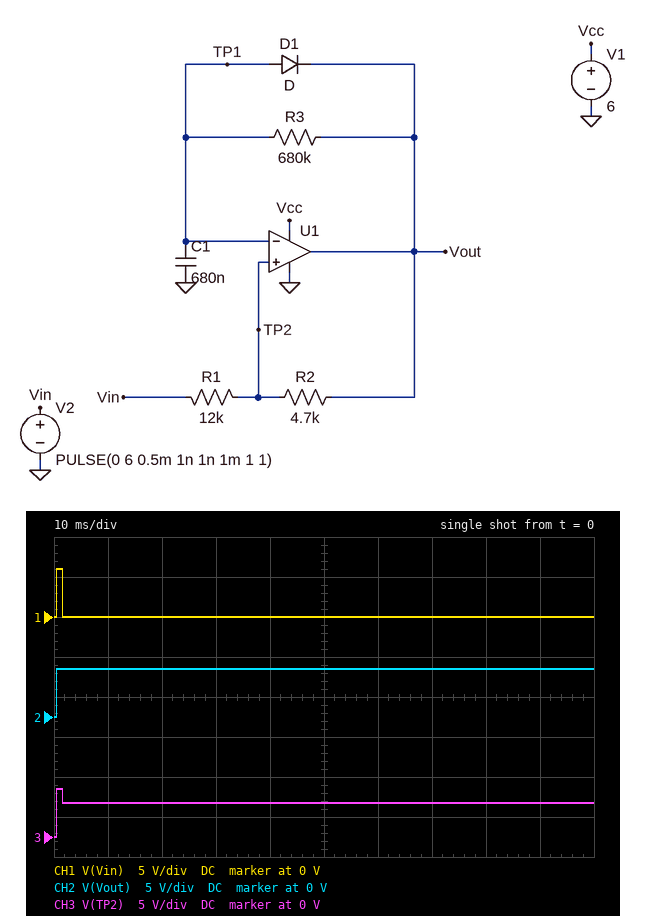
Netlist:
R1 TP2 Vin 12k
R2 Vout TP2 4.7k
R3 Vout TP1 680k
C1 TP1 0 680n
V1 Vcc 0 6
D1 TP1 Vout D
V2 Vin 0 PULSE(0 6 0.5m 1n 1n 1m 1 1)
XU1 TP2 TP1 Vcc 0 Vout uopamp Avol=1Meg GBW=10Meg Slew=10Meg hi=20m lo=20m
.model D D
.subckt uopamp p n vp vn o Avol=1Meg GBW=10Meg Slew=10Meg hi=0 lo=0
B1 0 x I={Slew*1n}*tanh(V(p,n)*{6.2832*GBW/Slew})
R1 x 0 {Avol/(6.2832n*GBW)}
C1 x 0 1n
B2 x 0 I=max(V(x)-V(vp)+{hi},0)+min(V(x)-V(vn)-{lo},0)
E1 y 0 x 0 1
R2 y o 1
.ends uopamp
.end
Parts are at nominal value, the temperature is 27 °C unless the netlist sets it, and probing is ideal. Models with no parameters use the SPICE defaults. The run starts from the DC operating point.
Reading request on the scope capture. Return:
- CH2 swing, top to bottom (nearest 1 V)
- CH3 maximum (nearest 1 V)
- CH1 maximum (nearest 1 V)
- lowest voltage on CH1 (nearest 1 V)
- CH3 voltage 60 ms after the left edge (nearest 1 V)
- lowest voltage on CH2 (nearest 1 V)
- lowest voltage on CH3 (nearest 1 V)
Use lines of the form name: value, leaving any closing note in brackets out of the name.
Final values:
CH2 swing, top to bottom: 6 V
CH3 maximum: 6 V
CH1 maximum: 6 V
lowest voltage on CH1: 0 V
CH3 voltage 60 ms after the left edge: 4 V
lowest voltage on CH2: 0 V
lowest voltage on CH3: 0 V
